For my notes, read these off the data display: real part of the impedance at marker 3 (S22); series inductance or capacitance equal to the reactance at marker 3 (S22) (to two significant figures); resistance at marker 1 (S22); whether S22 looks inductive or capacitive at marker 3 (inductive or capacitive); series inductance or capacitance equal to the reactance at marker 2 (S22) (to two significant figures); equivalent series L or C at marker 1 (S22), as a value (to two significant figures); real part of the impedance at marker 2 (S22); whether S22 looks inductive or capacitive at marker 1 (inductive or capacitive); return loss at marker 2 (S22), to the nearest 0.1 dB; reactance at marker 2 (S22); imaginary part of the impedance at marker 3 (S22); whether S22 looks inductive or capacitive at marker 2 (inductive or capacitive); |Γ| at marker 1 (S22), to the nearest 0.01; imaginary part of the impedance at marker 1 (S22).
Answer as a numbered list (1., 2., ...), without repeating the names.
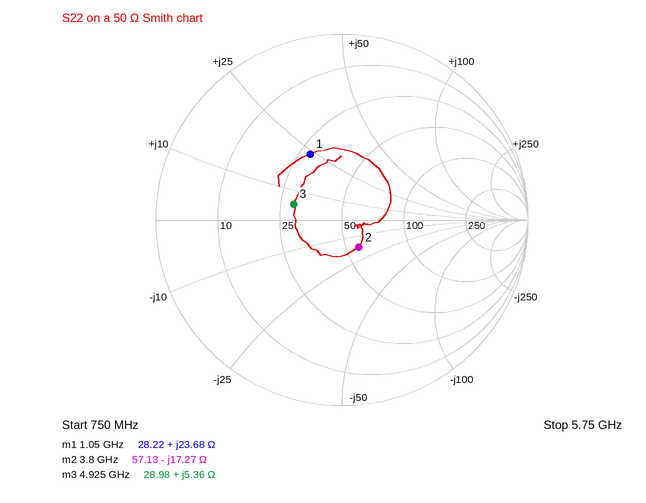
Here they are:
1. 28.98 Ω
2. 170 pH
3. 28.22 Ω
4. inductive
5. 2.4 pF
6. 3.6 nH
7. 57.13 Ω
8. inductive
9. 15.3 dB
10. -17.27 Ω
11. +5.36 Ω
12. capacitive
13. 0.39
14. +23.68 Ω
